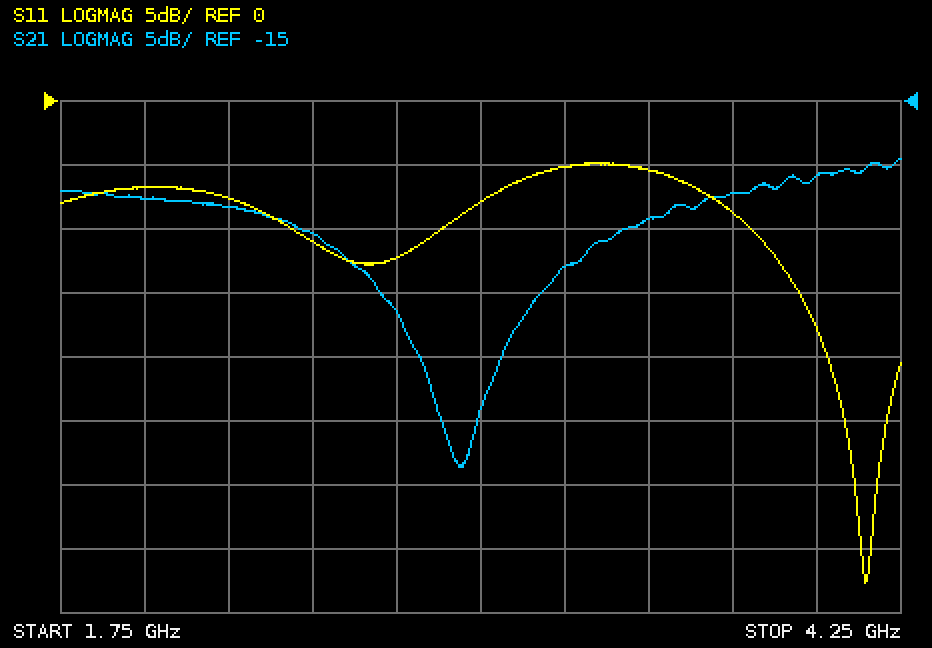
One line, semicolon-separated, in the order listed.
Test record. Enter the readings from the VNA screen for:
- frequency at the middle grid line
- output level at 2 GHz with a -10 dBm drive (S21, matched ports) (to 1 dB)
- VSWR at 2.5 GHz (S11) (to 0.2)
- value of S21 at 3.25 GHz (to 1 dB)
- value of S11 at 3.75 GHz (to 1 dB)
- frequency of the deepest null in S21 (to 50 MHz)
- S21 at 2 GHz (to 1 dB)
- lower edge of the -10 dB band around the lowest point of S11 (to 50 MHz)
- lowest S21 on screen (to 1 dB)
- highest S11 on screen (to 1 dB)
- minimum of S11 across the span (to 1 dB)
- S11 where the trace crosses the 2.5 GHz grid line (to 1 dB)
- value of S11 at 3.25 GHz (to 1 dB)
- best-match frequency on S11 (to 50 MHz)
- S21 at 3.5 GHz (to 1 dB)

3 GHz; -33 dBm; 1.8; -28 dB; -9 dB; 2.95 GHz; -23 dB; 3.80 GHz; -44 dB; -5 dB; -38 dB; -11 dB; -5 dB; 4.15 GHz; -24 dB
